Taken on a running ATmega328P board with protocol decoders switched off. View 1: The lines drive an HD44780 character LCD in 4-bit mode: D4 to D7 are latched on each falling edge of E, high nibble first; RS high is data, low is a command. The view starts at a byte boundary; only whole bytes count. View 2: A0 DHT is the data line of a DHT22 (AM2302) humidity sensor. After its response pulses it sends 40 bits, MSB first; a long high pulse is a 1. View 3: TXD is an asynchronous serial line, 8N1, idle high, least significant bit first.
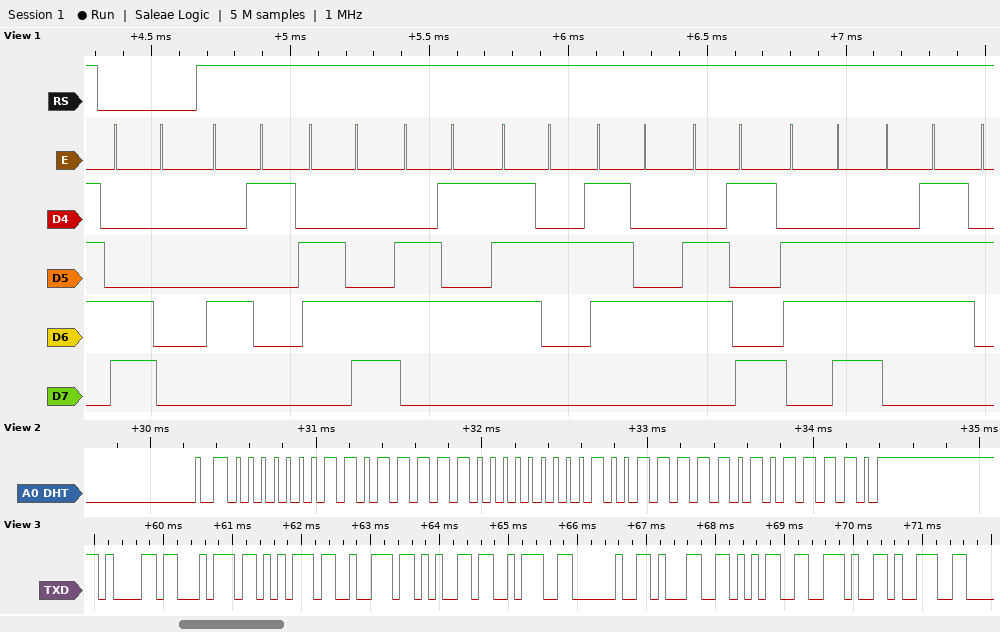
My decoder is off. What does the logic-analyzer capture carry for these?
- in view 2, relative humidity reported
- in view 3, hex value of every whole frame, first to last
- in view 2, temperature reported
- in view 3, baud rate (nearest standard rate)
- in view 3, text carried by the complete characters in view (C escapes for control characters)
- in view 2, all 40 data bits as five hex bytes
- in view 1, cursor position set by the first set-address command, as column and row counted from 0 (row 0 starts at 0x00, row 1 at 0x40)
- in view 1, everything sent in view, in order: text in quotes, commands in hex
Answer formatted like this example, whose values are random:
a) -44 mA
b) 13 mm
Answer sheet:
a) 44.6 %
b) 61 74 75 72 65 3A 20 31 35 2E 39
c) 15.9 °C
d) 9600 baud
e) "ature: 15.9"
f) 01 BE 00 9F 5E
g) column 0, row 1
h) 0xC0 "Alerting"
